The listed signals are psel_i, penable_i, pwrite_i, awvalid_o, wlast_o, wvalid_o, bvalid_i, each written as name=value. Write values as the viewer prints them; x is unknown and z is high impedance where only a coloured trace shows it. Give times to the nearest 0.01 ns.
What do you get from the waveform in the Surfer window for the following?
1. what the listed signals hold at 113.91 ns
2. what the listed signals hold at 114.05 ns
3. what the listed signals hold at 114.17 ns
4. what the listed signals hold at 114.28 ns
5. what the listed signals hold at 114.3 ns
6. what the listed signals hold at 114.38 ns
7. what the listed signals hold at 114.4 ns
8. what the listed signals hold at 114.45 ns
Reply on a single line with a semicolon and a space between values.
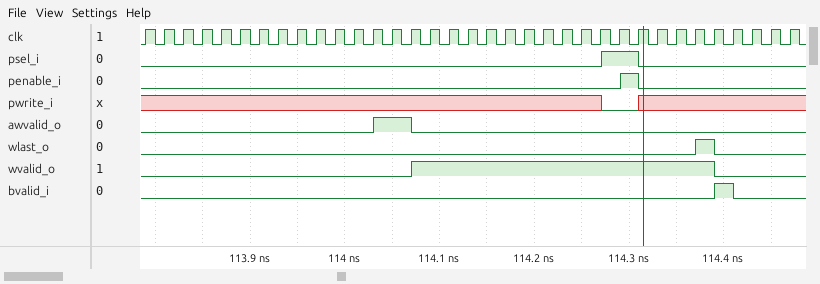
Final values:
psel_i=0, penable_i=0, pwrite_i=x, awvalid_o=0, wlast_o=0, wvalid_o=0, bvalid_i=0; psel_i=0, penable_i=0, pwrite_i=x, awvalid_o=1, wlast_o=0, wvalid_o=0, bvalid_i=0; psel_i=0, penable_i=0, pwrite_i=x, awvalid_o=0, wlast_o=0, wvalid_o=1, bvalid_i=0; psel_i=1, penable_i=0, pwrite_i=0, awvalid_o=0, wlast_o=0, wvalid_o=1, bvalid_i=0; psel_i=1, penable_i=1, pwrite_i=0, awvalid_o=0, wlast_o=0, wvalid_o=1, bvalid_i=0; psel_i=0, penable_i=0, pwrite_i=x, awvalid_o=0, wlast_o=1, wvalid_o=1, bvalid_i=0; psel_i=0, penable_i=0, pwrite_i=x, awvalid_o=0, wlast_o=0, wvalid_o=0, bvalid_i=1; psel_i=0, penable_i=0, pwrite_i=x, awvalid_o=0, wlast_o=0, wvalid_o=0, bvalid_i=0
